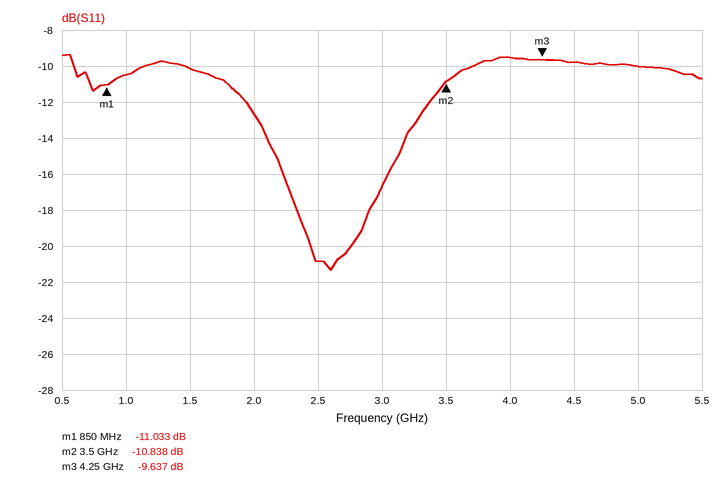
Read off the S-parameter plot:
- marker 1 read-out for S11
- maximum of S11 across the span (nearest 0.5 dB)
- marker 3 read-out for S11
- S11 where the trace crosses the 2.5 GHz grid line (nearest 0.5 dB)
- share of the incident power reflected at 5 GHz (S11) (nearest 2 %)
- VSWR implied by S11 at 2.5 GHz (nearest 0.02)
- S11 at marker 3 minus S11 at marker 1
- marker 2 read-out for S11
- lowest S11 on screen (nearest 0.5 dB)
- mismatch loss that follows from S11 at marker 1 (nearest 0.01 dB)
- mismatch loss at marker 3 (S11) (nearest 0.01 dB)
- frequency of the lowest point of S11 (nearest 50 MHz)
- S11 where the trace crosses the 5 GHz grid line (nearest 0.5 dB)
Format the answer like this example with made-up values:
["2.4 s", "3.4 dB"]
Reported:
["-11.033 dB", "-9.5 dB", "-9.637 dB", "-21.0 dB", "10 %", "1.20", "1.396 dB", "-10.838 dB", "-21.5 dB", "0.36 dB", "0.50 dB", "2.60 GHz", "-10.0 dB"]
